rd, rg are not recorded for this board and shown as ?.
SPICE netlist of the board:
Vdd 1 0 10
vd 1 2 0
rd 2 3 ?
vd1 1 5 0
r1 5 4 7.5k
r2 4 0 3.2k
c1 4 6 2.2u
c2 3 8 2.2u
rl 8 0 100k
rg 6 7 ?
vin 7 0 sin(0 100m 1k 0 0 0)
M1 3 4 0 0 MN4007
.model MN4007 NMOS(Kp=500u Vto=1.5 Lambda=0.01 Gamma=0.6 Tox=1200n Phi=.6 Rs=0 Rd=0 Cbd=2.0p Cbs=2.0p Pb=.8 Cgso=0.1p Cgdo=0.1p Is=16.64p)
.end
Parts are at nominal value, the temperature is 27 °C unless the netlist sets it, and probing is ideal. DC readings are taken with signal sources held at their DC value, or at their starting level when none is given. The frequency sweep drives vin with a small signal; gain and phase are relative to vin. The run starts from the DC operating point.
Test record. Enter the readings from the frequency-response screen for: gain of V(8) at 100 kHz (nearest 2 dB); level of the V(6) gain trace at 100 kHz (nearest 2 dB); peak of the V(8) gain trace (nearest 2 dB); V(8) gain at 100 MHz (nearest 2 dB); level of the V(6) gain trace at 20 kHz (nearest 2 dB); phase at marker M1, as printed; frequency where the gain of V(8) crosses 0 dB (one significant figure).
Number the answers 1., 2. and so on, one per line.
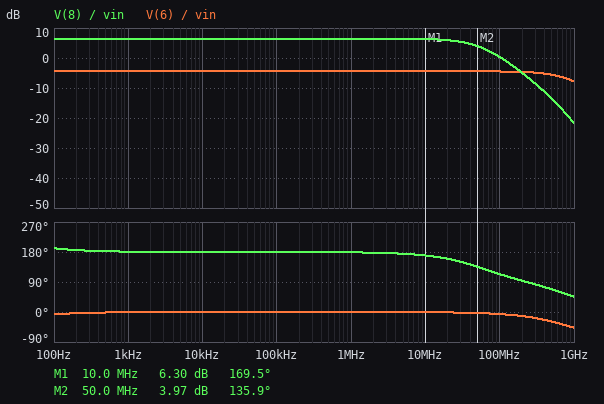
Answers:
1. 6 dB
2. -4 dB
3. 6 dB
4. 0 dB
5. -4 dB
6. 169.5 deg
7. 100 MHz
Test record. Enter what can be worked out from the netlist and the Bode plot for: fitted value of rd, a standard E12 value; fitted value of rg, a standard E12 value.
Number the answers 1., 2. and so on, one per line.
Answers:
1. 4.7 kΩ
2. 1.5 kΩ
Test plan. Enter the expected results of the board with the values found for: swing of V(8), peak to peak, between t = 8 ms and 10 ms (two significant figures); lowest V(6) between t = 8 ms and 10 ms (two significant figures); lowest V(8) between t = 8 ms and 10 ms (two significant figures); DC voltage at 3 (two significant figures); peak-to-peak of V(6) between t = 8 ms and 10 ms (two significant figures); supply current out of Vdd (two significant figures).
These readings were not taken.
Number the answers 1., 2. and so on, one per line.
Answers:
1. 420 mV
2. -60 mV
3. -210 mV
4. 7.2 V
5. 120 mV
6. 1.5 mA
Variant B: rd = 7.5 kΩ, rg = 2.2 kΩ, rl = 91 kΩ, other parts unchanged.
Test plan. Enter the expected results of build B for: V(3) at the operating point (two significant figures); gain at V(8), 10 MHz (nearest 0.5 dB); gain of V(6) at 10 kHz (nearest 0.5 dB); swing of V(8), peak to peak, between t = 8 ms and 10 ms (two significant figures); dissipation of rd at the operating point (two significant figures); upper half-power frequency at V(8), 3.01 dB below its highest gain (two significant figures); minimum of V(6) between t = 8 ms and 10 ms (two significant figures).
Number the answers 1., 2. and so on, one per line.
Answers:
1. 5.6 V
2. 8.0 dB
3. -6.0 dB
4. 530 mV
5. 2.6 mW
6. 34 MHz
7. -50 mV
